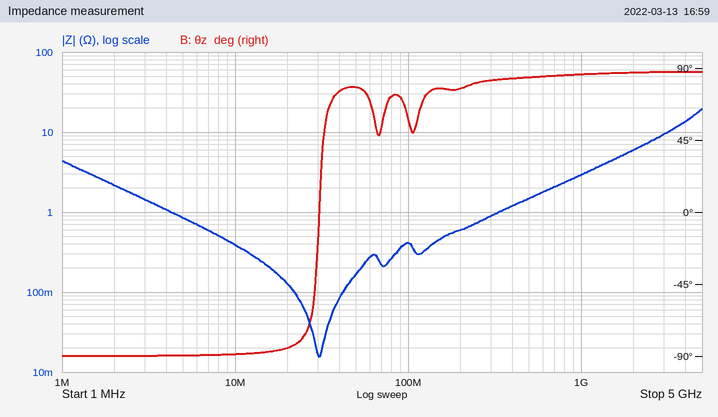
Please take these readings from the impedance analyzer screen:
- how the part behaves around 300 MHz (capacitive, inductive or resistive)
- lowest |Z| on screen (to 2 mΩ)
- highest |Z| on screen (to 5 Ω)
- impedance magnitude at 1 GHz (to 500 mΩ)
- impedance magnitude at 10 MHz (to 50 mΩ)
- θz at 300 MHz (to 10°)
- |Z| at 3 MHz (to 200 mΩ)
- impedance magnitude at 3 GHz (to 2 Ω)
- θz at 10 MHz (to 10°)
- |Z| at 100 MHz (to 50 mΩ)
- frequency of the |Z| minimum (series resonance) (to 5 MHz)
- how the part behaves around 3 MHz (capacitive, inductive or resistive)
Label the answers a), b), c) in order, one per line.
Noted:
a) inductive
b) 16 mΩ
c) 20 Ω
d) 3.0 Ω
e) 400 mΩ
f) 80°
g) 1.4 Ω
h) 10 Ω
i) -90°
j) 400 mΩ
k) 30 MHz
l) capacitive
